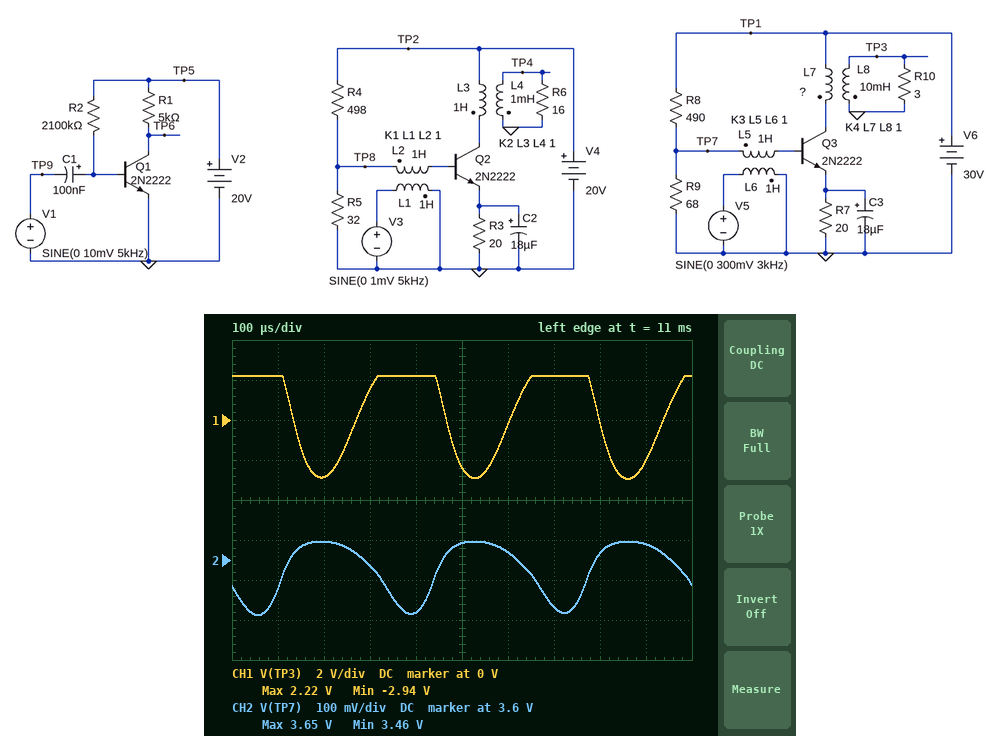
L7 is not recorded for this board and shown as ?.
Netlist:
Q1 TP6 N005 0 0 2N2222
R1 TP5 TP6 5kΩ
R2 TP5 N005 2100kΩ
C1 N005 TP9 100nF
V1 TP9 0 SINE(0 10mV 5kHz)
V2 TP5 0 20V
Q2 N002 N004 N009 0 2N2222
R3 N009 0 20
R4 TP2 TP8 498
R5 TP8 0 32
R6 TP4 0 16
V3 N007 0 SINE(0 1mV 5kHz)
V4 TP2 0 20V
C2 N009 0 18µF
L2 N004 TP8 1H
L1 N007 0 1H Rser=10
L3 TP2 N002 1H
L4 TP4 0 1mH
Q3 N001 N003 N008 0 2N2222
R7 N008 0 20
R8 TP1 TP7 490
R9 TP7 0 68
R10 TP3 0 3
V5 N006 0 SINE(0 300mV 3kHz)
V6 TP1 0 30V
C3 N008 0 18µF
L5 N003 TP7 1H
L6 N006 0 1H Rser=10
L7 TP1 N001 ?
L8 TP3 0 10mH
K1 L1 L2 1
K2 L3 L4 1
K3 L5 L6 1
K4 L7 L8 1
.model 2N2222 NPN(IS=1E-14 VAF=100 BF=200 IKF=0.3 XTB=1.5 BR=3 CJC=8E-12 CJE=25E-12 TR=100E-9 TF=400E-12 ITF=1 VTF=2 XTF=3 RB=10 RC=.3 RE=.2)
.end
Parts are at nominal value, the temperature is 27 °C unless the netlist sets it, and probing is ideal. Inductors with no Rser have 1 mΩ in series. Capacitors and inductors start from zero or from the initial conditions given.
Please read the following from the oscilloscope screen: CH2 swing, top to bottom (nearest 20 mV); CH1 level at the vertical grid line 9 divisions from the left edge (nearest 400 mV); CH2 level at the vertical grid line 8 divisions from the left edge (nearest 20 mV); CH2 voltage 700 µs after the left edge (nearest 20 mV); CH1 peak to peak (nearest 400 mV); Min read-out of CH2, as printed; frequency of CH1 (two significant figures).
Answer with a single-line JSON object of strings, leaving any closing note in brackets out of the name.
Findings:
{"CH2 swing, top to bottom": "180 mV", "CH1 level at the vertical grid line 9 divisions from the left edge": "-2.0 V", "CH2 level at the vertical grid line 8 divisions from the left edge": "3.62 V", "CH2 voltage 700 µs after the left edge": "3.48 V", "CH1 peak to peak": "5.2 V", "Min read-out of CH2, as printed": "3.46 V", "frequency of CH1": "3.0 kHz"}
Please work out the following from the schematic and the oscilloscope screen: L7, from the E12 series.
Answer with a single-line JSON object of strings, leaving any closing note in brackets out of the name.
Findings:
{"L7, from the E12 series": "1.5 H"}
